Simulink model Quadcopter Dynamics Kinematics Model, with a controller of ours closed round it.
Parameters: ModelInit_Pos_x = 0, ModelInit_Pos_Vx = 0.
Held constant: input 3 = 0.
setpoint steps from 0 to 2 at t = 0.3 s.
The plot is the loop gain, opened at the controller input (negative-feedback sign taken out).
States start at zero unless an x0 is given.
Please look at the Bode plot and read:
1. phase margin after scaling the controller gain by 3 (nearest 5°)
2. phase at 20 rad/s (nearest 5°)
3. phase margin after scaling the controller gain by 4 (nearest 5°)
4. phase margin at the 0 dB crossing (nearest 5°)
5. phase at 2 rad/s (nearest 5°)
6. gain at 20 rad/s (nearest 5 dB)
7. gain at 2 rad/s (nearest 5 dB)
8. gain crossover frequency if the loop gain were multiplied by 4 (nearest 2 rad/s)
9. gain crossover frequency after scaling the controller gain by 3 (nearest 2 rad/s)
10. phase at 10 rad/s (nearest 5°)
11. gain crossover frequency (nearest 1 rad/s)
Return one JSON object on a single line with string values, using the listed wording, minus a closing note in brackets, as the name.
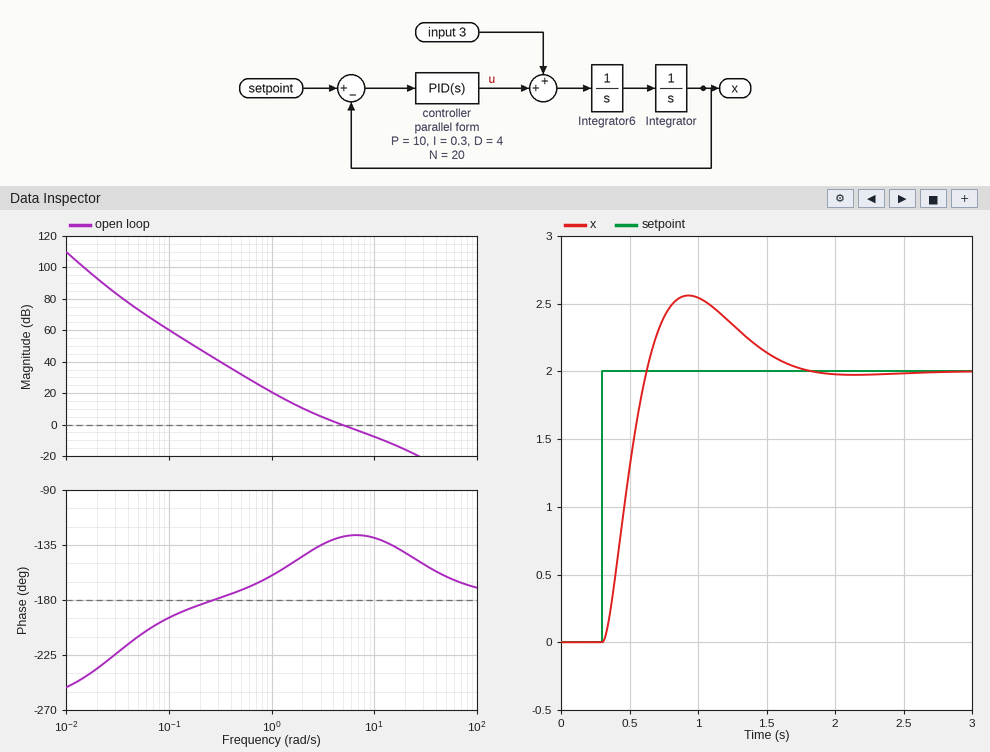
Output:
{"phase margin after scaling the controller gain by 3": "50°", "phase at 20 rad/s": "-140°", "phase margin after scaling the controller gain by 4": "45°", "phase margin at the 0 dB crossing": "50°", "phase at 2 rad/s": "-145°", "gain at 20 rad/s": "-15 dB", "gain at 2 rad/s": "10 dB", "gain crossover frequency if the loop gain were multiplied by 4": "14 rad/s", "gain crossover frequency after scaling the controller gain by 3": "12 rad/s", "phase at 10 rad/s": "-130°", "gain crossover frequency": "5 rad/s"}
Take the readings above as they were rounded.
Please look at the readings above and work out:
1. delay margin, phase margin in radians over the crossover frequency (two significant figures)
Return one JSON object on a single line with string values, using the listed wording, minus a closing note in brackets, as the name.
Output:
{"delay margin, phase margin in radians over the crossover frequency": "0.17 s"}
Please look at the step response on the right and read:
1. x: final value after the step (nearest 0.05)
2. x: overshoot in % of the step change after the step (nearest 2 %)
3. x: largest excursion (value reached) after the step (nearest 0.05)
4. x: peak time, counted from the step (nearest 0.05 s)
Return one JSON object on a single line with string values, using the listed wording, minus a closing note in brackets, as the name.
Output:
{"x: final value after the step": "2.00", "x: overshoot in % of the step change after the step": "28 %", "x: largest excursion (value reached) after the step": "2.55", "x: peak time, counted from the step": "0.65 s"}
